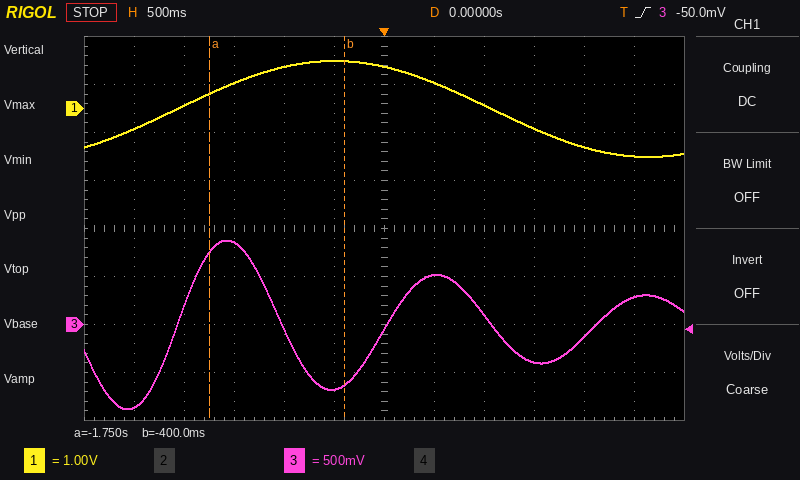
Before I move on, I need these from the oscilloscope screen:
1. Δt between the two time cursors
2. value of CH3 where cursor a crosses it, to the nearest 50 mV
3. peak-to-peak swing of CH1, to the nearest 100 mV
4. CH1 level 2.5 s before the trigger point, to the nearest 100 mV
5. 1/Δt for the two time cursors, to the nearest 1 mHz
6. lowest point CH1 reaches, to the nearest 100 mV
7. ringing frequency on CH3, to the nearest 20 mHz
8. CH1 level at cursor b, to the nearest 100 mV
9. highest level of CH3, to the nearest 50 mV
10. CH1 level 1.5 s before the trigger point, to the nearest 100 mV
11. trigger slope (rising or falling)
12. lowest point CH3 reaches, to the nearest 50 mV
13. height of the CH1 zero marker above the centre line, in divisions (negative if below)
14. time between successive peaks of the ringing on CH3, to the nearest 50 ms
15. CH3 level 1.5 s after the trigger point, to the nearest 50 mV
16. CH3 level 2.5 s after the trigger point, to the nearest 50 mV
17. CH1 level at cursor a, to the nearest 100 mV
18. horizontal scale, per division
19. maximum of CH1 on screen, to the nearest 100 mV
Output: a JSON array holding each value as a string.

["1.35 s", "750 mV", "2.0 V", "-400 mV", "741 mHz", "-1.0 V", "480 mHz", "1.0 V", "900 mV", "500 mV", "rising", "-900 mV", "+2.5 div", "2.10 s", "-400 mV", "300 mV", "300 mV", "500 ms", "1.0 V"]
